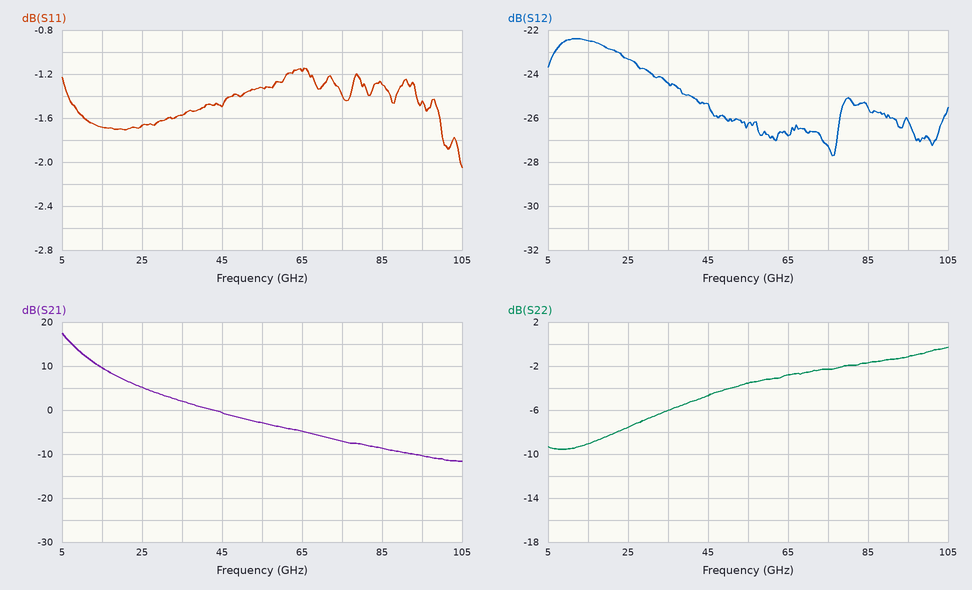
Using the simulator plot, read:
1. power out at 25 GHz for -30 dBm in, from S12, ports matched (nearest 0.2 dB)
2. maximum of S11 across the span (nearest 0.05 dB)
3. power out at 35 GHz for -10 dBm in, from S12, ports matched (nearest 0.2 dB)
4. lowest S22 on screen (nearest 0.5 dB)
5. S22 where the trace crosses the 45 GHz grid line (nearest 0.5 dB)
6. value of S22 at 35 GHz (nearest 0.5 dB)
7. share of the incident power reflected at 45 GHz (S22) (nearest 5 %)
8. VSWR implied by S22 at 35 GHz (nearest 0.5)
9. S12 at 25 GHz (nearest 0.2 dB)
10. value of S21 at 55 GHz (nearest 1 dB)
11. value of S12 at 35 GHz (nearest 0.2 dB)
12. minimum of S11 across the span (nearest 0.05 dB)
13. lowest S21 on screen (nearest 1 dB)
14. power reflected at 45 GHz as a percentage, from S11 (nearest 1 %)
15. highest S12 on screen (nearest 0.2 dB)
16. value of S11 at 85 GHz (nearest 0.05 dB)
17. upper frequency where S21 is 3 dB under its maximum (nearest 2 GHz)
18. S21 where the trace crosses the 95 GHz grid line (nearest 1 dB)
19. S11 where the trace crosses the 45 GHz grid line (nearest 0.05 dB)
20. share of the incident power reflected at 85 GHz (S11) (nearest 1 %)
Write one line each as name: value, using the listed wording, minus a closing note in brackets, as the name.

power out at 25 GHz for -30 dBm in, from S12, ports matched: -53.4 dBm
maximum of S11 across the span: -1.15 dB
power out at 35 GHz for -10 dBm in, from S12, ports matched: -34.4 dBm
lowest S22 on screen: -9.5 dB
S22 where the trace crosses the 45 GHz grid line: -4.5 dB
value of S22 at 35 GHz: -6.0 dB
share of the incident power reflected at 45 GHz (S22): 35 %
VSWR implied by S22 at 35 GHz: 3.0
S12 at 25 GHz: -23.4 dB
value of S21 at 55 GHz: -3 dB
value of S12 at 35 GHz: -24.4 dB
minimum of S11 across the span: -2.05 dB
lowest S21 on screen: -12 dB
power reflected at 45 GHz as a percentage, from S11: 71 %
highest S12 on screen: -22.4 dB
value of S11 at 85 GHz: -1.30 dB
upper frequency where S21 is 3 dB under its maximum: 8 GHz
S21 where the trace crosses the 95 GHz grid line: -10 dB
S11 where the trace crosses the 45 GHz grid line: -1.50 dB
share of the incident power reflected at 85 GHz (S11): 74 %
